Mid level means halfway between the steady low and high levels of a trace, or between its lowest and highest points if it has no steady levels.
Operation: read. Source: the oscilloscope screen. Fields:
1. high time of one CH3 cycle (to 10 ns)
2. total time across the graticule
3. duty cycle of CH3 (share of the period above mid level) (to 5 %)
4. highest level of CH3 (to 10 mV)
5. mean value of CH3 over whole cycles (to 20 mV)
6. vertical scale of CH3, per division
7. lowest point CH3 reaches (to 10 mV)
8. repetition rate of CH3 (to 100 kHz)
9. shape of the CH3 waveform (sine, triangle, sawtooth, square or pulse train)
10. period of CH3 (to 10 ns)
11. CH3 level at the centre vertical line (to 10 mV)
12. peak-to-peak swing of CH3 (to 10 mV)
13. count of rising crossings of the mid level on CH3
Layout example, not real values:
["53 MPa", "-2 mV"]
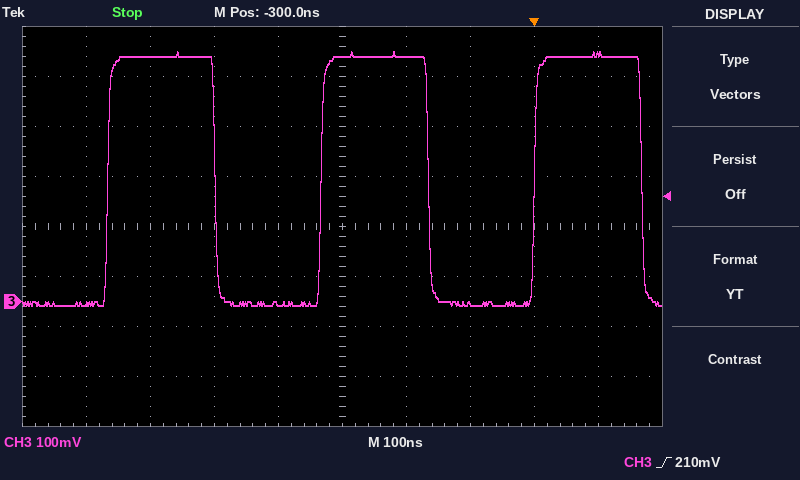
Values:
["170 ns", "1 µs", "50 %", "500 mV", "240 mV", "100 mV", "-10 mV", "3.0 MHz", "square", "330 ns", "490 mV", "510 mV", "3"]
